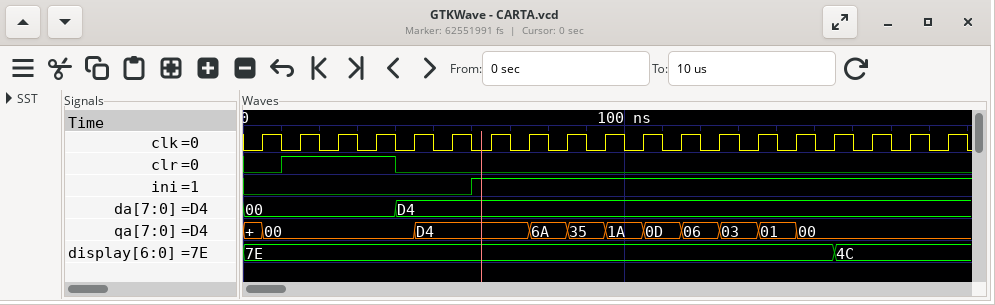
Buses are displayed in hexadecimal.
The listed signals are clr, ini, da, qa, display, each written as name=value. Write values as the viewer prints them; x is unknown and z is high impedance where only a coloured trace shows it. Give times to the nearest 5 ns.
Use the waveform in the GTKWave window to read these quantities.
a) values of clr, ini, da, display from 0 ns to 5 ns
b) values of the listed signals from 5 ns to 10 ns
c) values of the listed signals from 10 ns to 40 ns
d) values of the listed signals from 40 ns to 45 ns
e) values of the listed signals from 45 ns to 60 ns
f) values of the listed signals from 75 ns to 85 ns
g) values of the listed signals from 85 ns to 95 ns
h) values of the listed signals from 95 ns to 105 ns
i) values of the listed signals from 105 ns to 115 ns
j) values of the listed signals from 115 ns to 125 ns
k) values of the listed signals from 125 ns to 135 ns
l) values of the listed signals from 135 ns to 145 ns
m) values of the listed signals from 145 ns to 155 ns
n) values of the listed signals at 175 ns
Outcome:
clr=0, ini=0, da=00, display=7E
clr=0, ini=0, da=00, qa=00, display=7E
clr=1, ini=0, da=00, qa=00, display=7E
clr=0, ini=0, da=D4, qa=00, display=7E
clr=0, ini=0, da=D4, qa=D4, display=7E
clr=0, ini=1, da=D4, qa=6A, display=7E
clr=0, ini=1, da=D4, qa=35, display=7E
clr=0, ini=1, da=D4, qa=1A, display=7E
clr=0, ini=1, da=D4, qa=0D, display=7E
clr=0, ini=1, da=D4, qa=06, display=7E
clr=0, ini=1, da=D4, qa=03, display=7E
clr=0, ini=1, da=D4, qa=01, display=7E
clr=0, ini=1, da=D4, qa=00, display=7E
clr=0, ini=1, da=D4, qa=00, display=4C
